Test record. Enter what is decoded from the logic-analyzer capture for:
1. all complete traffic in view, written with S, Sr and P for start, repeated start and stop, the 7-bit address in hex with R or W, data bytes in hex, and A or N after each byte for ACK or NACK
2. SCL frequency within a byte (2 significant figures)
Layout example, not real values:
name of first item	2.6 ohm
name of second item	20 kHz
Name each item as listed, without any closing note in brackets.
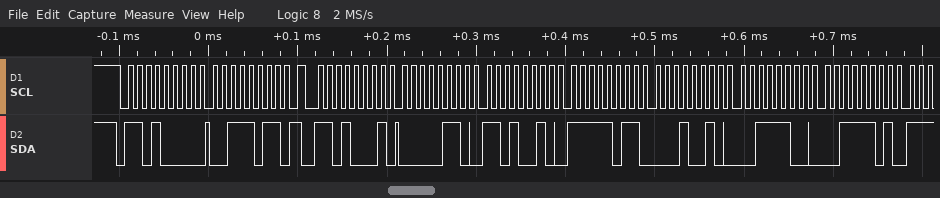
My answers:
all complete traffic in view, written with S, Sr and P for start, repeated start and stop, the 7-bit address in hex with R or W, data bytes in hex, and A or N after each byte for ACK or NACK	S 68W A 3B A Sr 68R A 06 A D2 A FB A 12 A 3C A 3D A
SCL frequency within a byte	100 kHz
